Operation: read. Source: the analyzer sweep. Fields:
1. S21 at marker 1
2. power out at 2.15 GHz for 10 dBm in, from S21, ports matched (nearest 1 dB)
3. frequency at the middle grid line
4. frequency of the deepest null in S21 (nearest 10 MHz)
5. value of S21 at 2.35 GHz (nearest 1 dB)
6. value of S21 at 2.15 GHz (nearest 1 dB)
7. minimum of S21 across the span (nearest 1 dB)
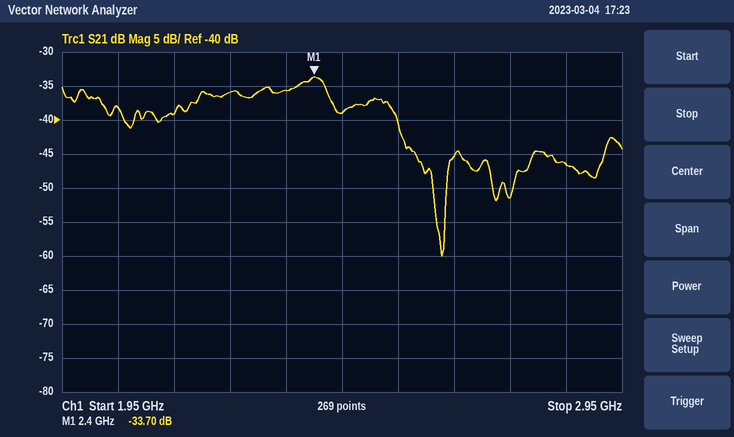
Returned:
-33.70 dB
-29 dBm
2.45 GHz
2.63 GHz
-36 dB
-39 dB
-60 dB
